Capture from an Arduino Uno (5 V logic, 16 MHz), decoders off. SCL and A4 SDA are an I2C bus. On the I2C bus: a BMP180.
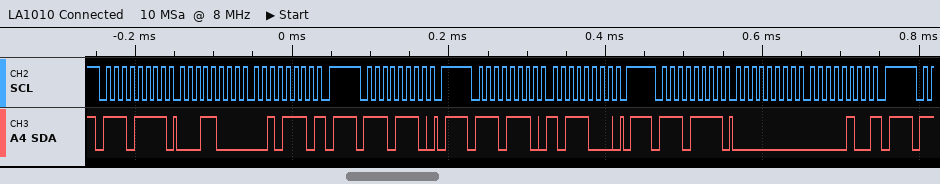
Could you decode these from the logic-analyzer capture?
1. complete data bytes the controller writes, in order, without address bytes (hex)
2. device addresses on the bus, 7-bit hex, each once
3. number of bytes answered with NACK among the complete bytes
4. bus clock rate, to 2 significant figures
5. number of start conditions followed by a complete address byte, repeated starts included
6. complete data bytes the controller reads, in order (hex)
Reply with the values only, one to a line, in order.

B8
0x77
2
100 kHz
4
18 2E 00 04
